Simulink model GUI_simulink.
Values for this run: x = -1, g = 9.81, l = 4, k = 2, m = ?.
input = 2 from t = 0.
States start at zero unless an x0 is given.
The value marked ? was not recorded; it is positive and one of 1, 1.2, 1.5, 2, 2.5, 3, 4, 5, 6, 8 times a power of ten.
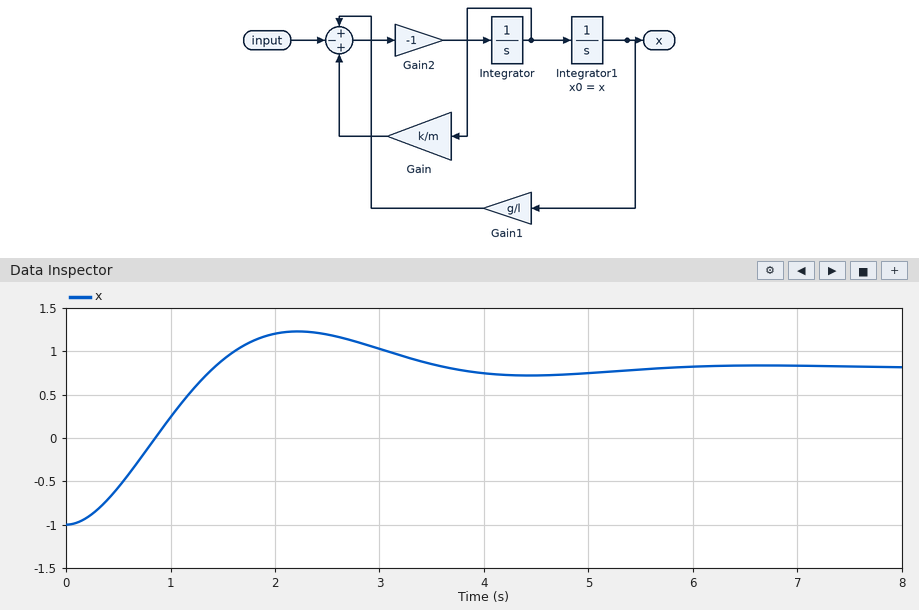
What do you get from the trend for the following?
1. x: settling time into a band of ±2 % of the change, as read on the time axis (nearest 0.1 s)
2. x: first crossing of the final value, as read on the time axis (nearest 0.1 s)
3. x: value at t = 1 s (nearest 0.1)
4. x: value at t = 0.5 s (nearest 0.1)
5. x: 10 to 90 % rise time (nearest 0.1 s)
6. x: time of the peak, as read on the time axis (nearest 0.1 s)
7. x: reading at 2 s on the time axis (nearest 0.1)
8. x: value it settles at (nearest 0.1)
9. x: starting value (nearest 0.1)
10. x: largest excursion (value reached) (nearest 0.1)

5.4 s
1.4 s
0.2
-0.6
1.0 s
2.2 s
1.2
0.8
-1.0
1.2
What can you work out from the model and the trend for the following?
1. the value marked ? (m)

1.5
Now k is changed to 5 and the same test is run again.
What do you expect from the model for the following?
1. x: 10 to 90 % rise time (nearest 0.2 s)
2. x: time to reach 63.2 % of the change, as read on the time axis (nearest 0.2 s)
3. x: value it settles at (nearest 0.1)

2.4 s
1.4 s
0.8
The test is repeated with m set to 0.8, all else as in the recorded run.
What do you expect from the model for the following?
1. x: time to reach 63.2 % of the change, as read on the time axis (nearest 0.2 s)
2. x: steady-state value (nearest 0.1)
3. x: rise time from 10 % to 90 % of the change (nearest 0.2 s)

1.2 s
0.8
1.6 s
